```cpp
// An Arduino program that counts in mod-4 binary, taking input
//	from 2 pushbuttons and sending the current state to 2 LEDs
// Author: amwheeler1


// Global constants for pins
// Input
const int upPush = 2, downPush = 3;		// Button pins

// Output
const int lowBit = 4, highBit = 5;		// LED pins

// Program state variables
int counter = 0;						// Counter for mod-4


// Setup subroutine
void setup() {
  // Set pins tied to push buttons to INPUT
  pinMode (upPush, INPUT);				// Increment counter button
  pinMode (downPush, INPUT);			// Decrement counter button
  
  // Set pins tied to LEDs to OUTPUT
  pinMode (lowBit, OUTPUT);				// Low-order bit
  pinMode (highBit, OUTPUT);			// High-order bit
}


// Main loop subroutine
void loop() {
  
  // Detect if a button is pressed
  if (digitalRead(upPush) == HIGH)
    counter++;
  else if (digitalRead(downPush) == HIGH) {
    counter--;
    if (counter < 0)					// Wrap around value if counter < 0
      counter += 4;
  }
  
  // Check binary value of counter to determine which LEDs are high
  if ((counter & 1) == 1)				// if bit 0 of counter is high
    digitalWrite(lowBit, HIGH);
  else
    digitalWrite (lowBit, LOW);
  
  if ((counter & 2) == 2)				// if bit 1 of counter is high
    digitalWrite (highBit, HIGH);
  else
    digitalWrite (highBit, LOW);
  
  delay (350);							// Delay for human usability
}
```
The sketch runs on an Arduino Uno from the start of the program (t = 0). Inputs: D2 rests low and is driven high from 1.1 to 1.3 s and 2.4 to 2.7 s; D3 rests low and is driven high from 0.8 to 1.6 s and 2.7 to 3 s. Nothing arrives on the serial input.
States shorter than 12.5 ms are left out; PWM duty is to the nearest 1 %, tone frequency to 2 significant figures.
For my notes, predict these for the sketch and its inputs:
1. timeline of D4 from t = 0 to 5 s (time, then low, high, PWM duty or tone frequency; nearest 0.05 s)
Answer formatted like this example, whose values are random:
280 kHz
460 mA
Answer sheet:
0 s low; 1.05 s high; 1.4 s low; 2.45 s high; 2.8 s low
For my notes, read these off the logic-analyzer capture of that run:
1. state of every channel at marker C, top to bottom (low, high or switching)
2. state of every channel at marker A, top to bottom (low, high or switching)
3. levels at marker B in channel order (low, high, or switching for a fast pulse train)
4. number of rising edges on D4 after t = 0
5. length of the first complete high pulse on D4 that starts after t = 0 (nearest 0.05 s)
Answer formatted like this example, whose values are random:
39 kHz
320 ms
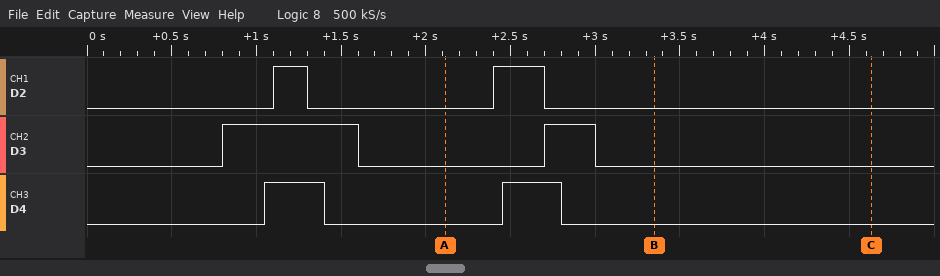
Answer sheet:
D2 low, D3 low, D4 low
D2 low, D3 low, D4 low
D2 low, D3 low, D4 low
2
0.35 s
